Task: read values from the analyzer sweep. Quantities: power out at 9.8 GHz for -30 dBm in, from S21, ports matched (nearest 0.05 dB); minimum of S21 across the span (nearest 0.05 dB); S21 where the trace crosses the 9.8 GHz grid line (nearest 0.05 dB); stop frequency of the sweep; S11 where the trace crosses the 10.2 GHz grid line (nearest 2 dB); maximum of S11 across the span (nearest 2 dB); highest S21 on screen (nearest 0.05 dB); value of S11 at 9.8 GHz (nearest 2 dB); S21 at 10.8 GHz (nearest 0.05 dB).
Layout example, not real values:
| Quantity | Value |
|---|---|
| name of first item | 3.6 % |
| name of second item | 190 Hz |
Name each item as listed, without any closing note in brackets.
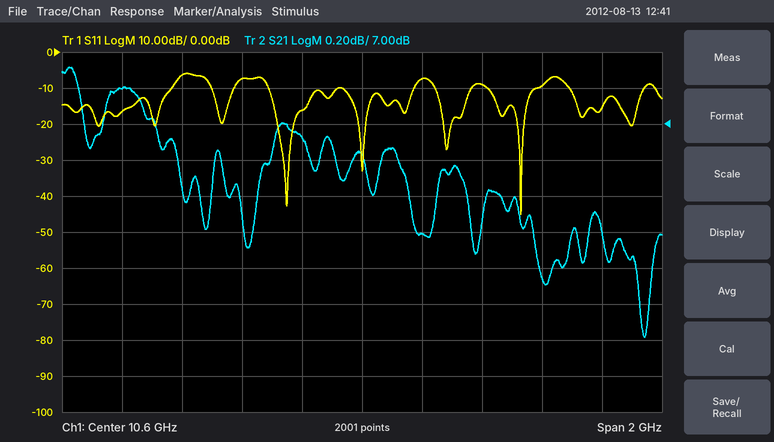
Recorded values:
| Quantity | Value |
|---|---|
| power out at 9.8 GHz for -30 dBm in, from S21, ports matched | -22.80 dBm |
| minimum of S21 across the span | 5.80 dB |
| S21 where the trace crosses the 9.8 GHz grid line | 7.20 dB |
| stop frequency of the sweep | 11.6 GHz |
| S11 where the trace crosses the 10.2 GHz grid line | -8 dB |
| maximum of S11 across the span | -6 dB |
| highest S21 on screen | 7.30 dB |
| value of S11 at 9.8 GHz | -16 dB |
| S21 at 10.8 GHz | 6.40 dB |
